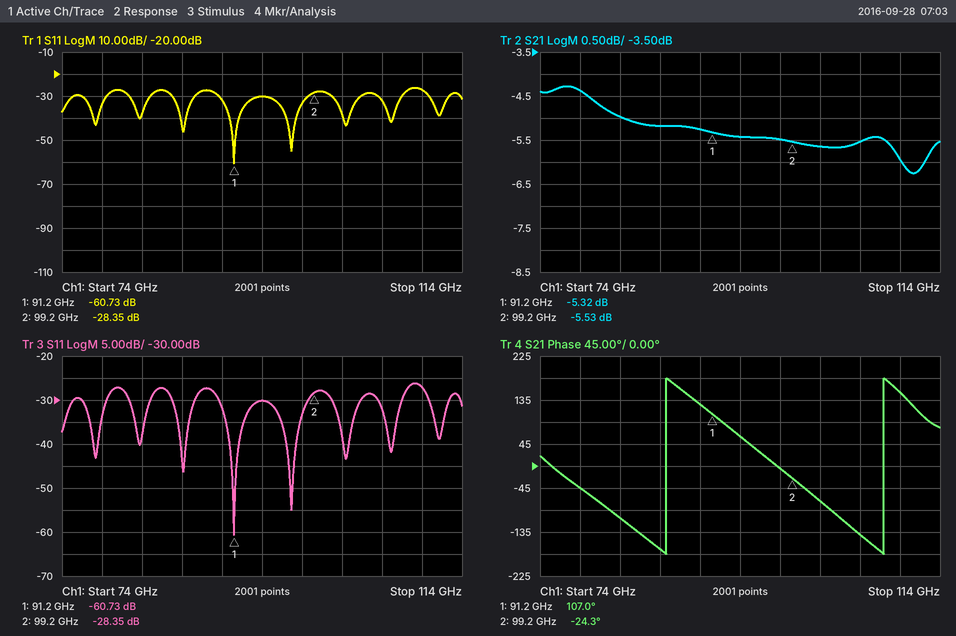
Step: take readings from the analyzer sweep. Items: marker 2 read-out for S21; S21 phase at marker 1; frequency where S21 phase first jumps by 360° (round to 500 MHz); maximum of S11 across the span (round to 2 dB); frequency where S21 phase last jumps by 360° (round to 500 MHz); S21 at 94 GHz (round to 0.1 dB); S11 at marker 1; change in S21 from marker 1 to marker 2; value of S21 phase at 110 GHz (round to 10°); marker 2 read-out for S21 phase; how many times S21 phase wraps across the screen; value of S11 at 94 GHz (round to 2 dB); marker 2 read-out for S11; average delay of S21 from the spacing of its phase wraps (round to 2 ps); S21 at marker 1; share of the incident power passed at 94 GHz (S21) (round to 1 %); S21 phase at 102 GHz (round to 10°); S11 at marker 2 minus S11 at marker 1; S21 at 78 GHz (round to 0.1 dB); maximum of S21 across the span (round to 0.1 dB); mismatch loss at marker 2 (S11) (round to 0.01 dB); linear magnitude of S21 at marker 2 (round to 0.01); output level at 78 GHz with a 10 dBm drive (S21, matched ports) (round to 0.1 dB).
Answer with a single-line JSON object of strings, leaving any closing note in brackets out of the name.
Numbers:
{"marker 2 read-out for S21": "-5.53 dB", "S21 phase at marker 1": "107.0°", "frequency where S21 phase first jumps by 360°": "86.5 GHz", "maximum of S11 across the span": "-26 dB", "frequency where S21 phase last jumps by 360°": "108.5 GHz", "S21 at 94 GHz": "-5.4 dB", "S11 at marker 1": "-60.73 dB", "change in S21 from marker 1 to marker 2": "-0.21 dB", "value of S21 phase at 110 GHz": "150°", "marker 2 read-out for S21 phase": "-24.3°", "how many times S21 phase wraps across the screen": "2", "value of S11 at 94 GHz": "-30 dB", "marker 2 read-out for S11": "-28.35 dB", "average delay of S21 from the spacing of its phase wraps": "46 ps", "S21 at marker 1": "-5.32 dB", "share of the incident power passed at 94 GHz (S21)": "29 %", "S21 phase at 102 GHz": "-70°", "S11 at marker 2 minus S11 at marker 1": "32.38 dB", "S21 at 78 GHz": "-4.4 dB", "maximum of S21 across the span": "-4.3 dB", "mismatch loss at marker 2 (S11)": "0.01 dB", "linear magnitude of S21 at marker 2": "0.53", "output level at 78 GHz with a 10 dBm drive (S21, matched ports)": "5.6 dBm"}
